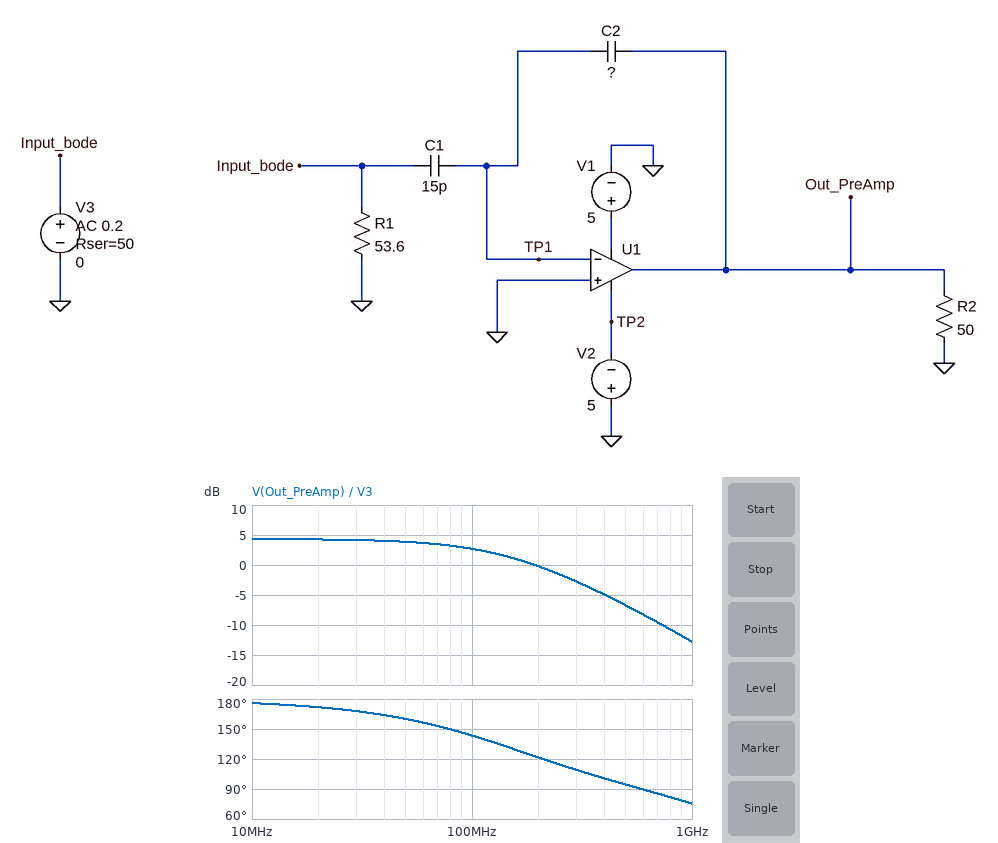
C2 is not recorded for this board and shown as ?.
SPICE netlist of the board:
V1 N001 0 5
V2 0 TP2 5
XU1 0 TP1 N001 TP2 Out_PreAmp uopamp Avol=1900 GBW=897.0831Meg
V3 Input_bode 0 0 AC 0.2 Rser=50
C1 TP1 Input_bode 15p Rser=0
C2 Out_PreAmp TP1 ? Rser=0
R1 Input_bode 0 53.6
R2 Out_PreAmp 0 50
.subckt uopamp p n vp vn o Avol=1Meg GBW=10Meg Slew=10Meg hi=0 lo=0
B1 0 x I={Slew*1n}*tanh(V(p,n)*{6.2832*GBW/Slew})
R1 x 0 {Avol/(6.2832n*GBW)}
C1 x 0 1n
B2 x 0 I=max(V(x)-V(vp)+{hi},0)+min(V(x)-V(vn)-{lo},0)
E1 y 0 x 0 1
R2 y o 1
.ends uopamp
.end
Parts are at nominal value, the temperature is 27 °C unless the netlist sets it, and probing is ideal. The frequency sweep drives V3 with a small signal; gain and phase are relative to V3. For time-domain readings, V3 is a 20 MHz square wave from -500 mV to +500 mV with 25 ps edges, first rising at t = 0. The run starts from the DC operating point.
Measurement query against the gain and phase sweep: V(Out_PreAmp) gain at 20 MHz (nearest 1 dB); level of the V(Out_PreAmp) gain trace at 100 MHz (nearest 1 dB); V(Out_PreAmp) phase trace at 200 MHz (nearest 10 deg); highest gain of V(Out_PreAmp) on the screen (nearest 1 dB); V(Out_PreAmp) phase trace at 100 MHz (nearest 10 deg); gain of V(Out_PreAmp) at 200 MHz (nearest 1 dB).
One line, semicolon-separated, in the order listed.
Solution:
4 dB; 3 dB; 120 deg; 4 dB; 140 deg; 0 dB
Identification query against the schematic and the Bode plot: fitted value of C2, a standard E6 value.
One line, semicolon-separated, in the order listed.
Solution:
4.7 pF
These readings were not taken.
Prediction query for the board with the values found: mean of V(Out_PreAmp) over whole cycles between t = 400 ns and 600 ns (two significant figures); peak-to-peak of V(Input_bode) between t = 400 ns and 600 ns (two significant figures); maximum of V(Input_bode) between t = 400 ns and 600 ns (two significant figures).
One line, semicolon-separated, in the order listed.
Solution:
-120 mV; 520 mV; 260 mV
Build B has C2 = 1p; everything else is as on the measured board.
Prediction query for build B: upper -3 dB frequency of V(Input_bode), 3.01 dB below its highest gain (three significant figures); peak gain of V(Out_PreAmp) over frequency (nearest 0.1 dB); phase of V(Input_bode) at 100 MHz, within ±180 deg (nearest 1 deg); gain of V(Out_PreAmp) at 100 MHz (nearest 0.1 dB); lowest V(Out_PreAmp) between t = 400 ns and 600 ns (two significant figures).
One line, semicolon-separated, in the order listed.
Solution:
5.41 GHz; 17.7 dB; -4 deg; 10.6 dB; -260 mV
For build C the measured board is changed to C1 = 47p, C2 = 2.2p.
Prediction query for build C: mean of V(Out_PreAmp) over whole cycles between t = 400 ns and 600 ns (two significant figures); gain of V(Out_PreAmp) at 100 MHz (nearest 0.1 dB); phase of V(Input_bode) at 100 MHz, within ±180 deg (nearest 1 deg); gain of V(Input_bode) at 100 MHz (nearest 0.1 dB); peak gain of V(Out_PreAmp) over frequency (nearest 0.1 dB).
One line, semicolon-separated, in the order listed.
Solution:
-140 mV; 10.2 dB; -6 deg; -7.7 dB; 20.8 dB
